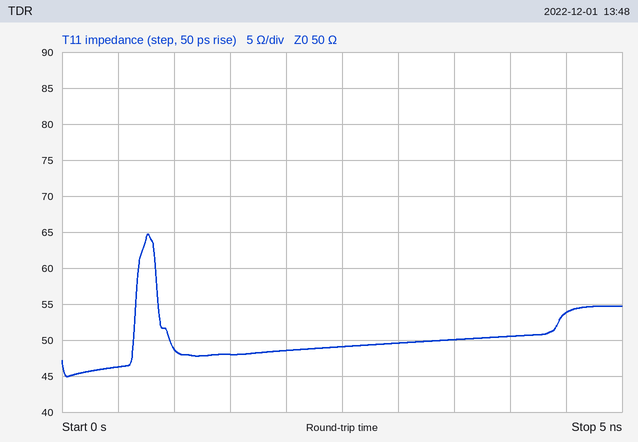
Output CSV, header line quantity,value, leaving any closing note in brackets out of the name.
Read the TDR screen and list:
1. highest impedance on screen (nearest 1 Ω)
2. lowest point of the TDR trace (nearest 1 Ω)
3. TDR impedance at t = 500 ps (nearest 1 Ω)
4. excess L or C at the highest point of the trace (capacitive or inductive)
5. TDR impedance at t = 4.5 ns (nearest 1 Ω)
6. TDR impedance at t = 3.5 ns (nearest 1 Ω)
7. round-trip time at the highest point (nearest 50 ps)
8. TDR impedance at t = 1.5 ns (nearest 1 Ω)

quantity,value
highest impedance on screen,65 Ω
lowest point of the TDR trace,45 Ω
TDR impedance at t = 500 ps,46 Ω
excess L or C at the highest point of the trace,inductive
TDR impedance at t = 4.5 ns,54 Ω
TDR impedance at t = 3.5 ns,50 Ω
round-trip time at the highest point,750 ps
TDR impedance at t = 1.5 ns,48 Ω
